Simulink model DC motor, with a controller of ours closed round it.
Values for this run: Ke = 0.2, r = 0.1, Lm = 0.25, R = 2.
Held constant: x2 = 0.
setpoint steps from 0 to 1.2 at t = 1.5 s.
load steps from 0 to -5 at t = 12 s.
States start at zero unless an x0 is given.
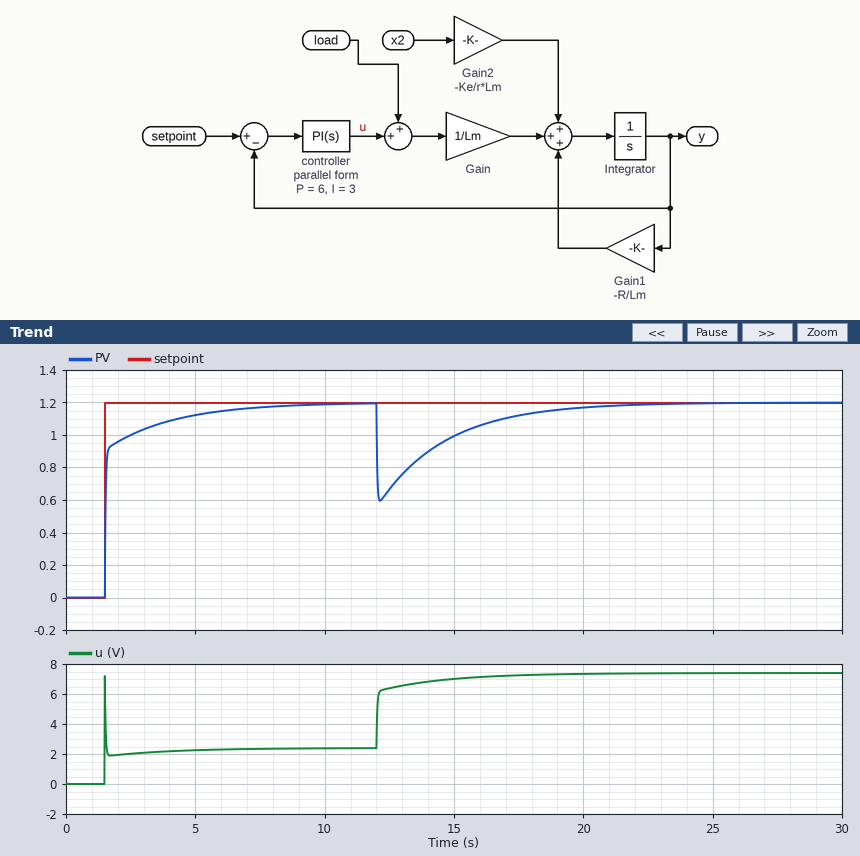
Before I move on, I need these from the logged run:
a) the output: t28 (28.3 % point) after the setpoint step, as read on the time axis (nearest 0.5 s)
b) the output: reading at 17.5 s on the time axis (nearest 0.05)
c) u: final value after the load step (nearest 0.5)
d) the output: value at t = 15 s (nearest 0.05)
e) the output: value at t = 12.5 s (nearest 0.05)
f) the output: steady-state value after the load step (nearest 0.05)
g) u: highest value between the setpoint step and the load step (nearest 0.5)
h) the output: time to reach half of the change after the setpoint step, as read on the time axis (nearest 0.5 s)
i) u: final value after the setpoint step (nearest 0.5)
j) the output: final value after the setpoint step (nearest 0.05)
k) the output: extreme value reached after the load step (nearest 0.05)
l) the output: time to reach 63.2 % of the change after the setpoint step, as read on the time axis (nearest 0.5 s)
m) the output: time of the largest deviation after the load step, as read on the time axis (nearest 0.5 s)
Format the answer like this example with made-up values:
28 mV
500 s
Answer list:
1.5 s
1.10
7.5
1.00
0.65
1.20
7.0
1.5 s
2.5
1.20
0.60
1.5 s
12.0 s
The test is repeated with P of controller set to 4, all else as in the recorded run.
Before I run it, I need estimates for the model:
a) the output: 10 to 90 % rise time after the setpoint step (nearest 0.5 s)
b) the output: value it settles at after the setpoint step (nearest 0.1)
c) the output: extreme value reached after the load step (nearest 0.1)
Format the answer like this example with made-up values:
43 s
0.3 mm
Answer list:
2.5 s
1.2
0.4
